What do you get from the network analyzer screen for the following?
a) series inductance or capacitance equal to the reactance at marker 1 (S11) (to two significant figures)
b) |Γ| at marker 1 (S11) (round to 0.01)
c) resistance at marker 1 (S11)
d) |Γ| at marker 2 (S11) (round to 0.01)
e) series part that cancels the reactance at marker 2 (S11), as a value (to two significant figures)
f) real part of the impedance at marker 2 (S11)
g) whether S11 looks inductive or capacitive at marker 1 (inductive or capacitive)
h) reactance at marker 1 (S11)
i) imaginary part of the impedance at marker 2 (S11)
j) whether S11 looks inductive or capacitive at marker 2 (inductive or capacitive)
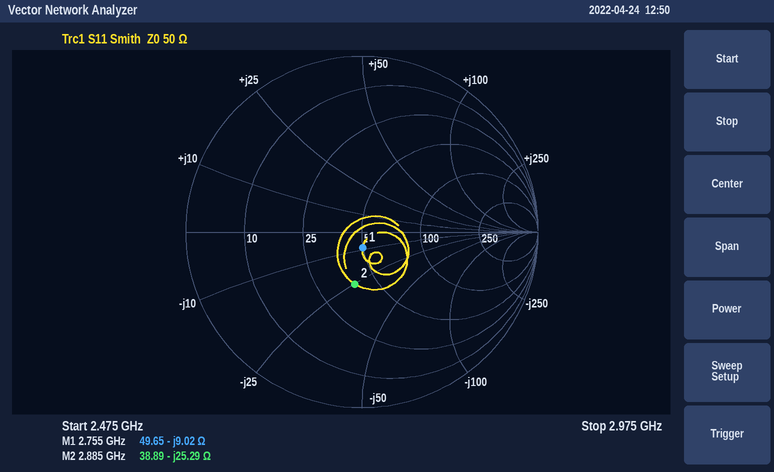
6.4 pF
0.09
49.65 Ω
0.30
1.4 nH
38.89 Ω
capacitive
-9.02 Ω
-25.29 Ω
capacitive
